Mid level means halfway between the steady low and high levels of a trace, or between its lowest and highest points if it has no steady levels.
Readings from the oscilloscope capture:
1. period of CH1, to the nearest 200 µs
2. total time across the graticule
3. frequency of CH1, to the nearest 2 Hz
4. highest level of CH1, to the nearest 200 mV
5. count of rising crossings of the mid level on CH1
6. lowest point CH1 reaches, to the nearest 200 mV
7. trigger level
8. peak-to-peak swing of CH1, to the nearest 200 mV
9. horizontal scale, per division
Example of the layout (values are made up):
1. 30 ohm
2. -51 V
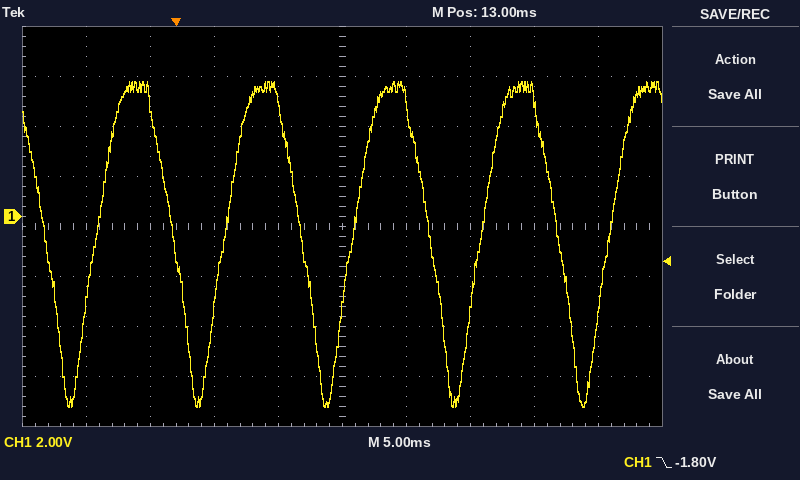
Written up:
1. 10.0 ms
2. 50 ms
3. 100 Hz
4. 5.4 V
5. 5
6. -7.6 V
7. -1.80 V
8. 13.0 V
9. 5 ms
